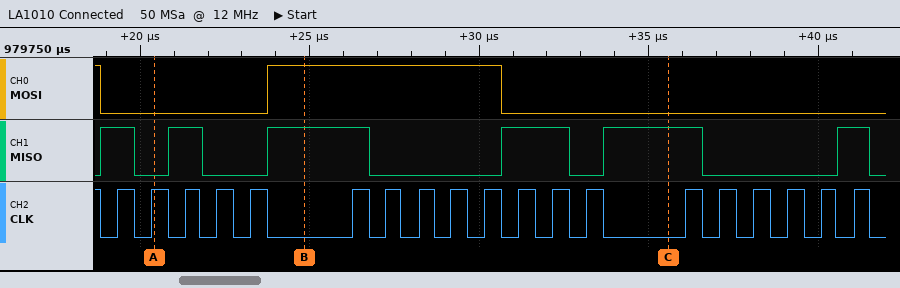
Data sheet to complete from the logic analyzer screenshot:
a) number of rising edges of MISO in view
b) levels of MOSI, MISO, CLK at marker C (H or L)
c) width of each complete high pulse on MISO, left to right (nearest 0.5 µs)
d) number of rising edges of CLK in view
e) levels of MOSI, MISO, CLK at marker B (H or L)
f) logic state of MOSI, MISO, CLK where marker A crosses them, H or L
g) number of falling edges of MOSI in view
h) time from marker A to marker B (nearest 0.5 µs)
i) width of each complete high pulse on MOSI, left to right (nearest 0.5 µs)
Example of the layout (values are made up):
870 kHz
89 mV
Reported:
6
MOSI=L, MISO=H, CLK=L
1 µs, 1 µs, 3 µs, 2 µs, 3 µs, 1 µs
19
MOSI=H, MISO=H, CLK=L
MOSI=L, MISO=L, CLK=H
2
4.5 µs
7 µs
